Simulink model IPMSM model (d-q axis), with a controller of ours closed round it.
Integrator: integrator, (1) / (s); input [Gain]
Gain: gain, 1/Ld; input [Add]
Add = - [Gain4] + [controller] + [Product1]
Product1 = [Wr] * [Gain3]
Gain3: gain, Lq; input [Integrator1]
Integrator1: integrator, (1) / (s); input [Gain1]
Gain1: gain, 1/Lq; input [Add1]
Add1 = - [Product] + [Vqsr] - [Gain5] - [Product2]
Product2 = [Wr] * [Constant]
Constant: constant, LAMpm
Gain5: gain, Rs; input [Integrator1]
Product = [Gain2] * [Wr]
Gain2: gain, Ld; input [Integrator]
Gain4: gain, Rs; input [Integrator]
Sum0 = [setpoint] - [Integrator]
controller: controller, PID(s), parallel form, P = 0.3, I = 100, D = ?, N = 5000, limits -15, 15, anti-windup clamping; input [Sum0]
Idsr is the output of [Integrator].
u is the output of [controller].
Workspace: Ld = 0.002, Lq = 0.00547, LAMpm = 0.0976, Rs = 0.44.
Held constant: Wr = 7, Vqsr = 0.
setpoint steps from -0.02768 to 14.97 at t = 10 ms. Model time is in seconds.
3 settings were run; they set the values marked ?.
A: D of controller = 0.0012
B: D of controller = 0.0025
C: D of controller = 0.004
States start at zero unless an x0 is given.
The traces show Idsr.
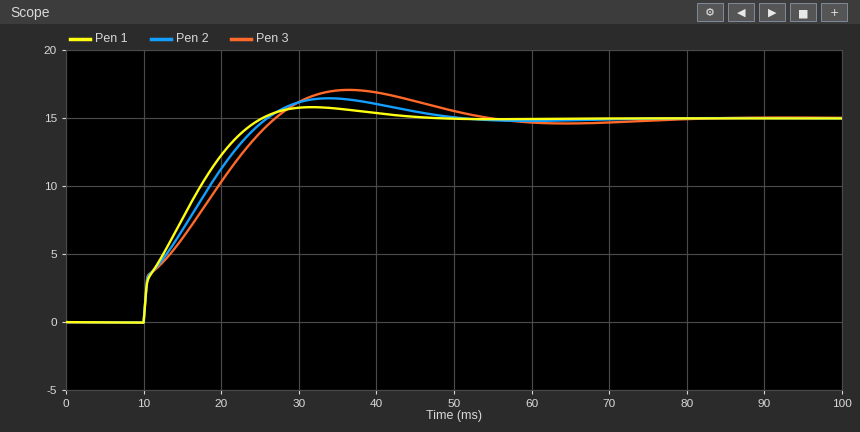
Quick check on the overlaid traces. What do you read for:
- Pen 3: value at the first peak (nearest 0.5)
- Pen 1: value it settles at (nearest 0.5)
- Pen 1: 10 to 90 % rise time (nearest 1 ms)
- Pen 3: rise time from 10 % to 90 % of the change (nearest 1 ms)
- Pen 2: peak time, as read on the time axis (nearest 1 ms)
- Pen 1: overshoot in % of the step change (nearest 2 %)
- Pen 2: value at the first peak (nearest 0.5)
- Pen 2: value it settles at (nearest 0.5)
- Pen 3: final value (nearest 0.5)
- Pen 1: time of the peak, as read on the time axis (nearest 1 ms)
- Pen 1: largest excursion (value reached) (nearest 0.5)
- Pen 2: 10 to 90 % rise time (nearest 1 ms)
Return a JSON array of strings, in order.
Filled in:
["17.0", "15.0", "12 ms", "14 ms", "34 ms", "6 %", "16.5", "15.0", "15.0", "32 ms", "16.0", "13 ms"]
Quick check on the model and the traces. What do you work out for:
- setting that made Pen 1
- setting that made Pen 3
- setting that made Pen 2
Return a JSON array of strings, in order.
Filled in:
["A", "C", "B"]
